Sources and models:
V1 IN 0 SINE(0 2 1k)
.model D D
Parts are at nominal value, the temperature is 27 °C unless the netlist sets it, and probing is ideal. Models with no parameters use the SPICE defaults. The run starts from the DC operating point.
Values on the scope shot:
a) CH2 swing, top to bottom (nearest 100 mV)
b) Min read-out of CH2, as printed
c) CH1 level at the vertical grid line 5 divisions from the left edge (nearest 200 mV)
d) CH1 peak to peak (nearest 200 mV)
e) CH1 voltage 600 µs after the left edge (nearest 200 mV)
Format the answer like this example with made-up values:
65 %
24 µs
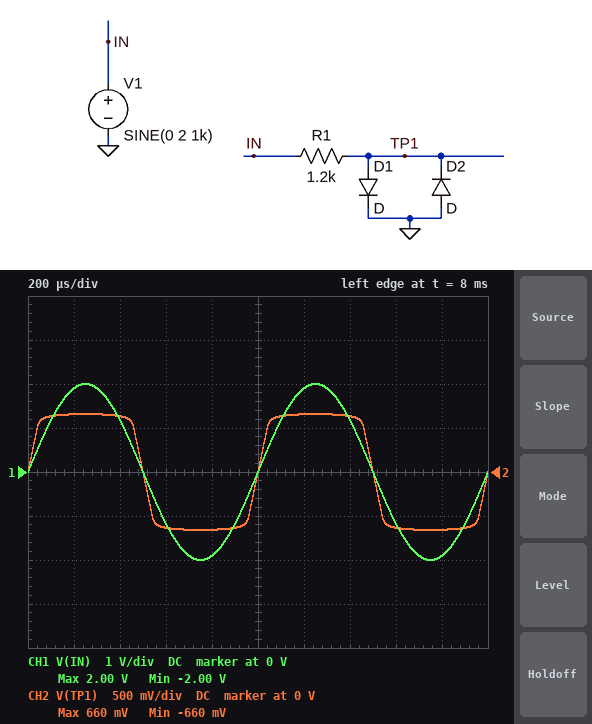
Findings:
1.3 V
-660 mV
0 V
4.0 V
-1.2 V
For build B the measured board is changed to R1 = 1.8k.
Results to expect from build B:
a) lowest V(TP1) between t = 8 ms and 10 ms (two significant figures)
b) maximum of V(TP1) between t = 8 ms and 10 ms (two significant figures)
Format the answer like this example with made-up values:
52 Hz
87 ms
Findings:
-650 mV
650 mV
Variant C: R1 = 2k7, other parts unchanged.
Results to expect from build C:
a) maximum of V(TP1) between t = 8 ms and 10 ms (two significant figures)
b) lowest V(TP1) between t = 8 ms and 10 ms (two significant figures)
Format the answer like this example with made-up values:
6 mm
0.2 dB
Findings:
640 mV
-640 mV
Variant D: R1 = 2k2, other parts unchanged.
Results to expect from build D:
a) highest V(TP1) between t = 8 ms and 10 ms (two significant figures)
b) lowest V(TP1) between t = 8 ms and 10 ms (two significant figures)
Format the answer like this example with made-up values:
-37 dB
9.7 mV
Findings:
640 mV
-640 mV
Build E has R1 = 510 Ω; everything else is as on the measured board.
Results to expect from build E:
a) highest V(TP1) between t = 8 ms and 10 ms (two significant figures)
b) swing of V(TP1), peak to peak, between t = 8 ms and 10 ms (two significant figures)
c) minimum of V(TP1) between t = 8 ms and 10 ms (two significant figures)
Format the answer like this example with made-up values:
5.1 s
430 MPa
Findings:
680 mV
1.4 V
-680 mV
